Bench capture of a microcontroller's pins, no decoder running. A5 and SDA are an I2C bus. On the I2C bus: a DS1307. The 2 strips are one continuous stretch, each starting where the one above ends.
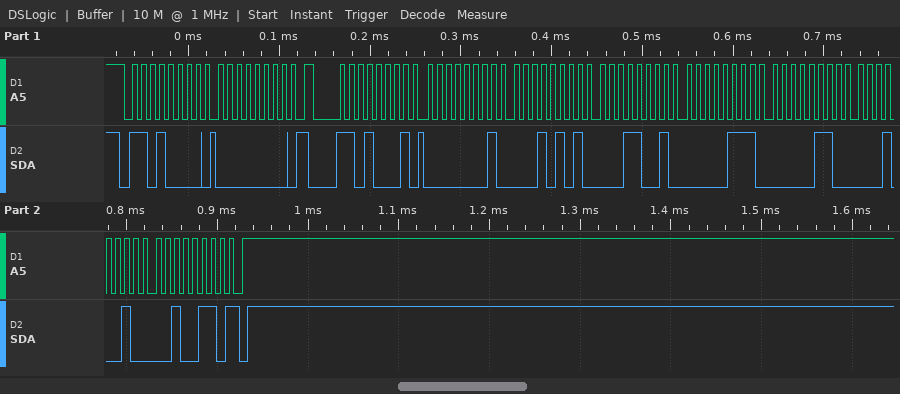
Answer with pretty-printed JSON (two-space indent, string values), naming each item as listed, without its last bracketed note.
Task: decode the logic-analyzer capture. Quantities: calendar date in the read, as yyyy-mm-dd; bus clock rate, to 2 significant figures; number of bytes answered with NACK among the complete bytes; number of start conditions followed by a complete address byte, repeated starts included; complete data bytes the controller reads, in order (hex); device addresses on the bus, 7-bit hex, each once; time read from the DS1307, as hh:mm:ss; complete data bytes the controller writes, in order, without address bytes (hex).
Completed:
{
  "calendar date in the read, as yyyy-mm-dd": "2026-12-06",
  "bus clock rate, to 2 significant figures": "100 kHz",
  "number of bytes answered with NACK among the complete bytes": "1",
  "number of start conditions followed by a complete address byte, repeated starts included": "2",
  "complete data bytes the controller reads, in order": "01 15 19 07 06 12 26",
  "device addresses on the bus, 7-bit hex, each once": "0x68",
  "time read from the DS1307, as hh:mm:ss": "19:15:01",
  "complete data bytes the controller writes, in order, without address bytes": "00"
}
